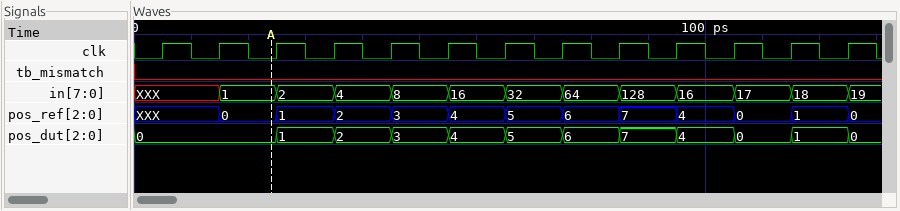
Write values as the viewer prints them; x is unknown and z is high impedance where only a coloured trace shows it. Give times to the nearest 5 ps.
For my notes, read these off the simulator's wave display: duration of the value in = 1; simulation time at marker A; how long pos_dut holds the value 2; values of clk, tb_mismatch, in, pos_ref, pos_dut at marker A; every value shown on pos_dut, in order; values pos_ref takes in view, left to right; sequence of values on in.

10 ps
25 ps
10 ps
clk=0, tb_mismatch=0, in=1, pos_ref=0, pos_dut=0
0, 1, 2, 3, 4, 5, 6, 7, 4, 0, 1, 0
XXX, 0, 1, 2, 3, 4, 5, 6, 7, 4, 0, 1, 0
XXX, 1, 2, 4, 8, 16, 32, 64, 128, 16, 17, 18, 19
